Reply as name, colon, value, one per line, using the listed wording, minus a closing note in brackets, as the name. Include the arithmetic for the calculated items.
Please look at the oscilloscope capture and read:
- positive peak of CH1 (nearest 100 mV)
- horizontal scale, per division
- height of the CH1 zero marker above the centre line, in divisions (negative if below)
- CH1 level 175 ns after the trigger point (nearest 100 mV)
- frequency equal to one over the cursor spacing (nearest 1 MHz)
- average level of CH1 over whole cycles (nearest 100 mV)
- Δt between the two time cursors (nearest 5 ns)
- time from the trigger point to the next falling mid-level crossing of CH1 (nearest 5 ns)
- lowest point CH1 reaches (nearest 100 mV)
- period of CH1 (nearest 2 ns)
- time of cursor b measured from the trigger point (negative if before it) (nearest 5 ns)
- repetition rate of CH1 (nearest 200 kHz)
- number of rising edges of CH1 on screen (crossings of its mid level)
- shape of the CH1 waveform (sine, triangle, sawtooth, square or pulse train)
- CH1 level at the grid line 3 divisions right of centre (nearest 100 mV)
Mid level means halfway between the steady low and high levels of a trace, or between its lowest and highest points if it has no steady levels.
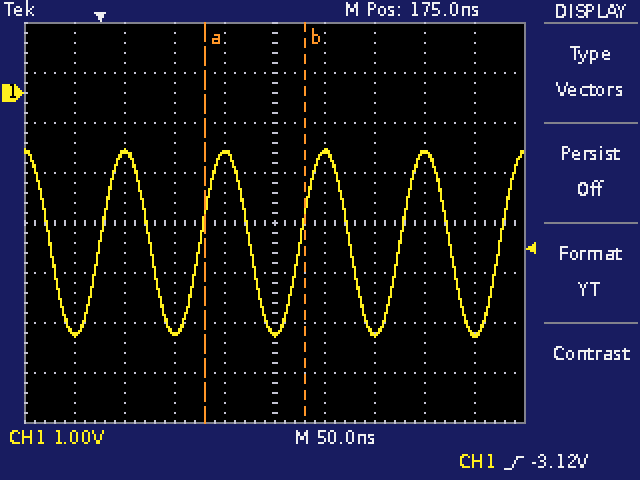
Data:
positive peak of CH1: -1.1 V
horizontal scale, per division: 50 ns
height of the CH1 zero marker above the centre line, in divisions: +2.6 div
CH1 level 175 ns after the trigger point: -4.8 V
frequency equal to one over the cursor spacing: 1 / 100 ns ≈ 10 MHz
average level of CH1 over whole cycles: (-1.1 V + (-4.9 V)) / 2 ≈ -3.0 V
Δt between the two time cursors: 100 ns
time from the trigger point to the next falling mid-level crossing of CH1: 50 ns
lowest point CH1 reaches: -4.9 V
period of CH1: 100 ns
time of cursor b measured from the trigger point (negative if before it): +205 ns
repetition rate of CH1: 1 / 100 ns ≈ 10.0 MHz
number of rising edges of CH1 on screen: 5
shape of the CH1 waveform: sine
CH1 level at the grid line 3 divisions right of centre: -1.2 V
